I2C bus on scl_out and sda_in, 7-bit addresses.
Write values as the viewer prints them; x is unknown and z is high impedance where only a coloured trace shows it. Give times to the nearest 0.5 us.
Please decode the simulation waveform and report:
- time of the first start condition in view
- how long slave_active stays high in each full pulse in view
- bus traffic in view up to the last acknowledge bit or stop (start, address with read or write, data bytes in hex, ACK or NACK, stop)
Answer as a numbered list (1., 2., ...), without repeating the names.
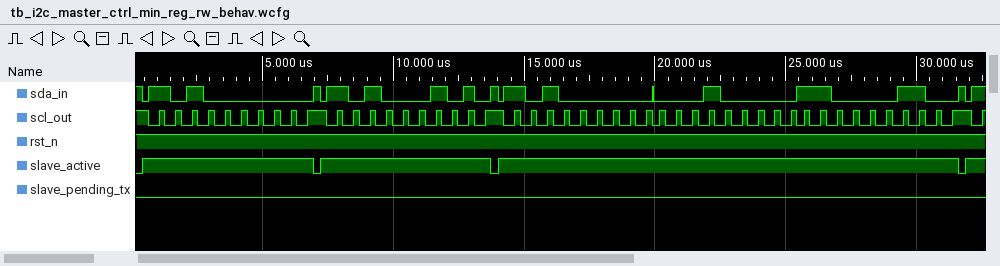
1. 0.5 us
2. 6.5 us, 6.5 us, 17.5 us
3. start, address 50 write ACK, stop, start, address 51 write NACK, stop, start, address 50 write ACK, 10 ACK, C3 ACK, stop
